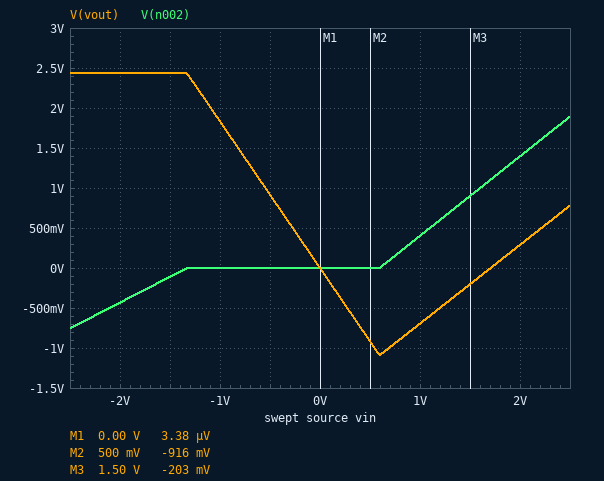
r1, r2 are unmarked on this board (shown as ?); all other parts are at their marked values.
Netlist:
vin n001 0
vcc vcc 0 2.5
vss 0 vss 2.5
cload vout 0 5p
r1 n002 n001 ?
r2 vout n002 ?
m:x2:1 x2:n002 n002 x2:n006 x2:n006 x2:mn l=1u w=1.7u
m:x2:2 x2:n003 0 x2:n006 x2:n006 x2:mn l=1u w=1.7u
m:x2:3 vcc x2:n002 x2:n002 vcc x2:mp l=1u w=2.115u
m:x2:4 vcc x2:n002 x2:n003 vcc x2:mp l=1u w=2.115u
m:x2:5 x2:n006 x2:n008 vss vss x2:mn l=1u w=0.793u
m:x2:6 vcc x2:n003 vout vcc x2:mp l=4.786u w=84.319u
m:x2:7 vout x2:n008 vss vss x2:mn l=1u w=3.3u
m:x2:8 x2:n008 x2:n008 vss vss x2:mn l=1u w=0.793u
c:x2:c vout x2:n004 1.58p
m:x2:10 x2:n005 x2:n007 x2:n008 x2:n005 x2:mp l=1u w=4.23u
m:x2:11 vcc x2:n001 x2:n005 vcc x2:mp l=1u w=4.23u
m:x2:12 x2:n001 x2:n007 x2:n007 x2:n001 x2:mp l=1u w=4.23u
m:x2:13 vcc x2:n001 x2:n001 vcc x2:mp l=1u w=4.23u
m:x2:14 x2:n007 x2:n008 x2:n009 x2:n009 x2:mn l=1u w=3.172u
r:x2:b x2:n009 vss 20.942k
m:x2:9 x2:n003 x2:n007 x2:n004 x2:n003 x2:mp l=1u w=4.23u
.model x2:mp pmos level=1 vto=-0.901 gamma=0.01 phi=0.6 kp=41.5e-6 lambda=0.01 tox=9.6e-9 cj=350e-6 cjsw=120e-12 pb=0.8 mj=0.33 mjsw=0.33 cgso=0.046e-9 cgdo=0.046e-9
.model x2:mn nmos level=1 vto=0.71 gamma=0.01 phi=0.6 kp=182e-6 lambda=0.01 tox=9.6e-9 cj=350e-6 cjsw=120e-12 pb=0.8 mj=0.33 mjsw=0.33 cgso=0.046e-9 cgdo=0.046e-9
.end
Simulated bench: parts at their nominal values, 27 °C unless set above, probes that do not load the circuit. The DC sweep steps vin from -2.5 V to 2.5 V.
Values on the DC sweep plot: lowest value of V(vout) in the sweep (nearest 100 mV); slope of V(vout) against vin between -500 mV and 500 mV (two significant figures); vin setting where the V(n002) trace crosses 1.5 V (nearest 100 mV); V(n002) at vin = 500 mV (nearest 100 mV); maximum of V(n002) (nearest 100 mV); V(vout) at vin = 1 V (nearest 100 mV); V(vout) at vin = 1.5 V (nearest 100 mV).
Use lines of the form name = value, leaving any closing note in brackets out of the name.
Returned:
lowest value of V(vout) in the sweep = -1.1 V
slope of V(vout) against vin between -500 mV and 500 mV = -1.8 V/V
vin setting where the V(n002) trace crosses 1.5 V = 2.1 V
V(n002) at vin = 500 mV = 0 V
maximum of V(n002) = 1.9 V
V(vout) at vin = 1 V = -700 mV
V(vout) at vin = 1.5 V = -200 mV
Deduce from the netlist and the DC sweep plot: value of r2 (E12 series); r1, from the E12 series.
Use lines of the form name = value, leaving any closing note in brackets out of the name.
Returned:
value of r2 = 33 kΩ
r1, from the E12 series = 18 kΩ
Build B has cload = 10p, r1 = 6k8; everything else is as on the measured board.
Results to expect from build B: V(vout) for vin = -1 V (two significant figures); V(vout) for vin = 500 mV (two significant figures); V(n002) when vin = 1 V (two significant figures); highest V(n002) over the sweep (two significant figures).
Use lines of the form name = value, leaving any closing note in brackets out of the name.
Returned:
V(vout) for vin = -1 V = 2.4 V
V(vout) for vin = 500 mV = -820 mV
V(n002) when vin = 1 V = 770 mV
highest V(n002) over the sweep = 2.3 V
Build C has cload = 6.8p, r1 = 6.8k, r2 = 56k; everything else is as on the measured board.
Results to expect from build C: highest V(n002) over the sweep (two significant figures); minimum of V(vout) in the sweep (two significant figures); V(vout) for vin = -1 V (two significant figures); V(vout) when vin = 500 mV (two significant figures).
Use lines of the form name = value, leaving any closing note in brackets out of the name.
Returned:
highest V(n002) over the sweep = 2.3 V
minimum of V(vout) in the sweep = -1.8 V
V(vout) for vin = -1 V = 2.5 V
V(vout) when vin = 500 mV = -1.6 V
